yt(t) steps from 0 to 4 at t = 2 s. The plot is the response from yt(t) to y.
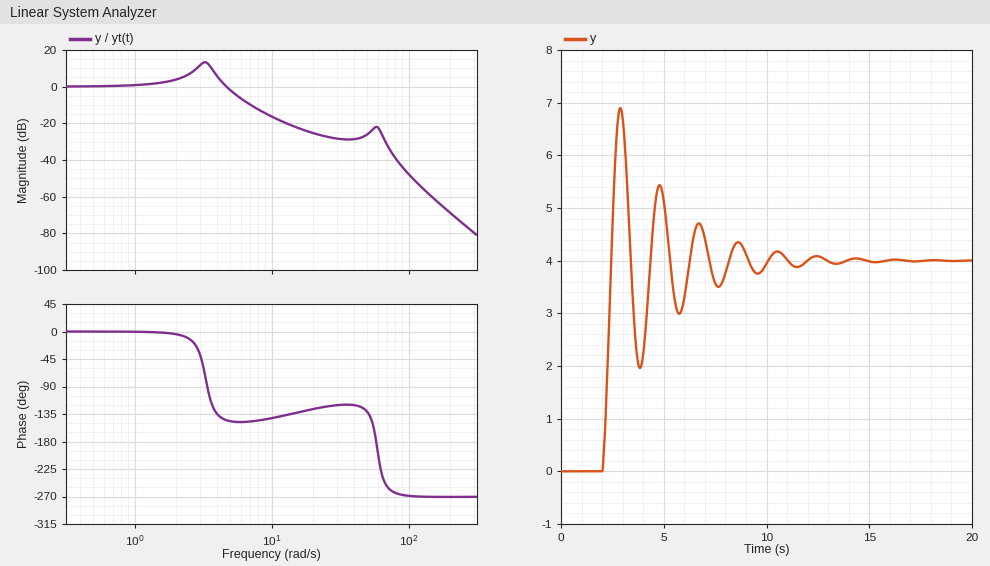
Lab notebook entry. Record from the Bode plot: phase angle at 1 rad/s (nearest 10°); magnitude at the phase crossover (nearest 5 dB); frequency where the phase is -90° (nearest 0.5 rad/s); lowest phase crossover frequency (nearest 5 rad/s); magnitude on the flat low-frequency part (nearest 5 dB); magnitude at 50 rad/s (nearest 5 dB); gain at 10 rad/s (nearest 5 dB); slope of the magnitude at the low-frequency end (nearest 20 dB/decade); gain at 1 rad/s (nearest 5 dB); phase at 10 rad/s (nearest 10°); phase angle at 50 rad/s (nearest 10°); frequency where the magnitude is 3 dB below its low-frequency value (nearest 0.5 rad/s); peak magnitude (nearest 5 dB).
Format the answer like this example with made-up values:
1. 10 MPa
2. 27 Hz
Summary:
1. 0°
2. -20 dB
3. 3.5 rad/s
4. 60 rad/s
5. 0 dB
6. -25 dB
7. -15 dB
8. 0 dB/decade
9. 0 dB
10. -140°
11. -130°
12. 5.0 rad/s
13. 15 dB
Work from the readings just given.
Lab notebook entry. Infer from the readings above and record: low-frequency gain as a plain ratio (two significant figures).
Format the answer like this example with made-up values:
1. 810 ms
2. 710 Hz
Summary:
1. 1.0
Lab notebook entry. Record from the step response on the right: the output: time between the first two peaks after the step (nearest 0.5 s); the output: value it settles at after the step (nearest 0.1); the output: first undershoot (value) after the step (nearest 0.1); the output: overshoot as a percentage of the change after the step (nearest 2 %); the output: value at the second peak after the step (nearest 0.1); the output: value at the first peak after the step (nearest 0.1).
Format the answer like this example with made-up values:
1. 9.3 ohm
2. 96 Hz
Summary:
1. 2.0 s
2. 4.0
3. 2.0
4. 72 %
5. 5.4
6. 6.9
